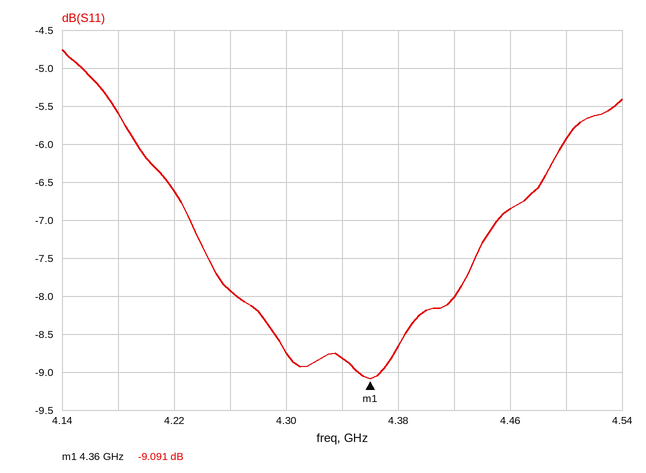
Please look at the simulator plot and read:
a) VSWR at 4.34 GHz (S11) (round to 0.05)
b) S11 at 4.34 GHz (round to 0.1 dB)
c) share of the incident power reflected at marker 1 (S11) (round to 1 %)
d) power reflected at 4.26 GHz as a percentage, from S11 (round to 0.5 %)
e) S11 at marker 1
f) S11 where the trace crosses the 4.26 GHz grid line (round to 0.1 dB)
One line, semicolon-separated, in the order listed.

2.15; -8.8 dB; 12 %; 16.0 %; -9.091 dB; -7.9 dB
